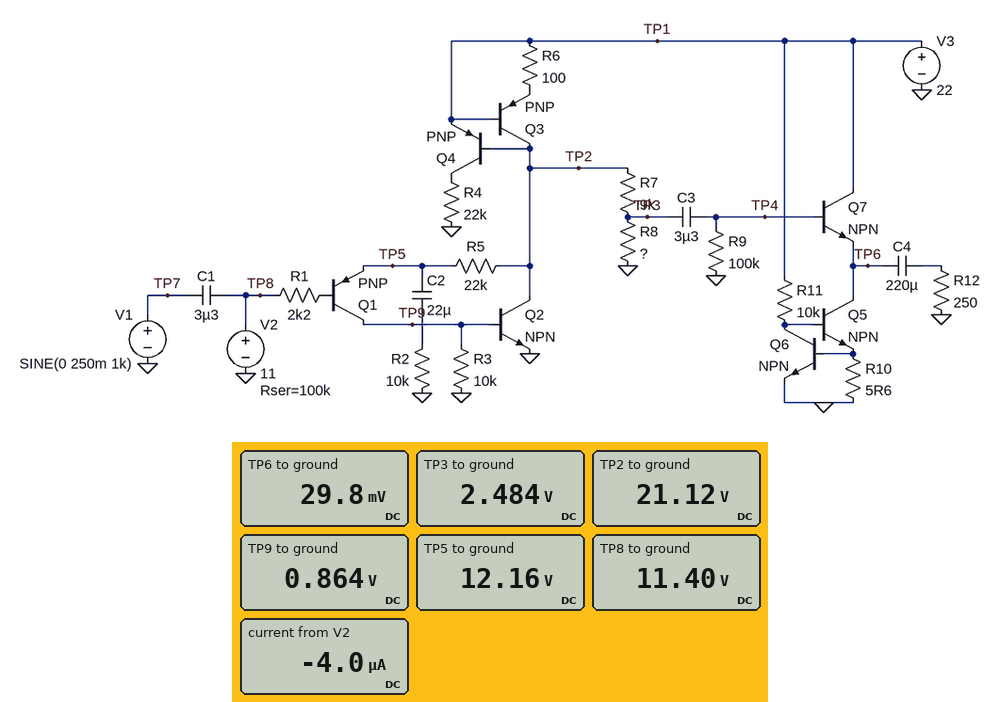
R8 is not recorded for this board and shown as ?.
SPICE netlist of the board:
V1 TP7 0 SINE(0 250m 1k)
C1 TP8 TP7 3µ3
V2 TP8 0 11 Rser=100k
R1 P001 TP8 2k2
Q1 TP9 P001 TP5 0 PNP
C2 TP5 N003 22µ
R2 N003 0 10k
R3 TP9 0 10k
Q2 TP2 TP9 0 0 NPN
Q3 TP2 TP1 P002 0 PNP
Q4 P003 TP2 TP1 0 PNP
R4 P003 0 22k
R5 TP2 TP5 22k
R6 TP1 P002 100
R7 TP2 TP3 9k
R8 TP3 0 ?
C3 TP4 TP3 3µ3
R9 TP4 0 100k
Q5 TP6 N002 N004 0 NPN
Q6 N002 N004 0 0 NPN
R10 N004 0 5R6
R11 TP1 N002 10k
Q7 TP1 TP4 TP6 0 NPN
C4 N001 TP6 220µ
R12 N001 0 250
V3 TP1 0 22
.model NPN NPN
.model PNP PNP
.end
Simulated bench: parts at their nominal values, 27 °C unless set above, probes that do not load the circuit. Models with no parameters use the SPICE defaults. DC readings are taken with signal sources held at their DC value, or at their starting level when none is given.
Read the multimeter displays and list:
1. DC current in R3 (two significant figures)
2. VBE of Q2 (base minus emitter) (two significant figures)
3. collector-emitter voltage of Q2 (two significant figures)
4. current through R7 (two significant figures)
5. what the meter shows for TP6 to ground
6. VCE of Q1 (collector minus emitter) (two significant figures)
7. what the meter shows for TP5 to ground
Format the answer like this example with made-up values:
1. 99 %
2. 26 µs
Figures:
1. 86 µA
2. 860 mV
3. 21 V
4. 2.1 mA
5. 29.8 mV
6. -11 V
7. 12.16 V
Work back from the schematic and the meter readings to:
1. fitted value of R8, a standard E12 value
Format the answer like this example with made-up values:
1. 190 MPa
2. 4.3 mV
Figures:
1. 1.2 kΩ
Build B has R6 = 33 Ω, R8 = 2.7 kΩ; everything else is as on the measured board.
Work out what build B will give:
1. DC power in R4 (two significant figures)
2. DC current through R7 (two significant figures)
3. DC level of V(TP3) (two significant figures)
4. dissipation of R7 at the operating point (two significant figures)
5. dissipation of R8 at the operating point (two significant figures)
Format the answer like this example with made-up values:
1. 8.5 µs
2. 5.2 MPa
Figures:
1. 22 mW
2. 1.8 mA
3. 4.9 V
4. 29 mW
5. 8.8 mW
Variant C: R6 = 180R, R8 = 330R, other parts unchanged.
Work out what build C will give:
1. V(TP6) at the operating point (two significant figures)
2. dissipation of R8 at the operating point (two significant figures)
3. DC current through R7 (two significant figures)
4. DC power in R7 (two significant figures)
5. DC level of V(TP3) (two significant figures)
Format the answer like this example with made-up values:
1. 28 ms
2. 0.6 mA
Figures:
1. 30 mV
2. 1.7 mW
3. 2.3 mA
4. 46 mW
5. 750 mV
